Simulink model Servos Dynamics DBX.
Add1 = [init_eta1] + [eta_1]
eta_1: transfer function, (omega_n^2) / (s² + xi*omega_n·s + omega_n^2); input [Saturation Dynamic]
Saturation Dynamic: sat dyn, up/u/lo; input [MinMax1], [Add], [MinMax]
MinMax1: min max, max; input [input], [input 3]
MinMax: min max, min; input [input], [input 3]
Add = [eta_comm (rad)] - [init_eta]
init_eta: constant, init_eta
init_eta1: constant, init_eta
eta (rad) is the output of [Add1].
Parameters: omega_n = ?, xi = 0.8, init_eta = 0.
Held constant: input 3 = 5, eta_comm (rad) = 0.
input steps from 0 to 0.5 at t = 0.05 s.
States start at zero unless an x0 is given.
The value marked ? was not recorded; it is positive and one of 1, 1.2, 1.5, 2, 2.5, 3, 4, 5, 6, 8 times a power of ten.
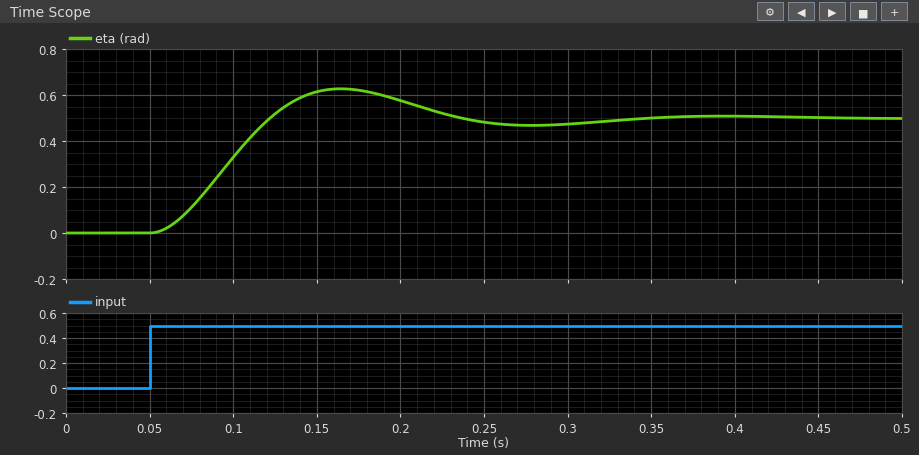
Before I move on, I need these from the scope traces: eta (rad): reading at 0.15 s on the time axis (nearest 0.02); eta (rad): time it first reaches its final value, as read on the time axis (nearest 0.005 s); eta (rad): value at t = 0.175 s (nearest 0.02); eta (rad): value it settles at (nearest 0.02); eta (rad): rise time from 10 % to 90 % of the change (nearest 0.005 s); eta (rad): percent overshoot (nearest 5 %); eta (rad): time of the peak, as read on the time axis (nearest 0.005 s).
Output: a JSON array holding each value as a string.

["0.62", "0.120 s", "0.62", "0.50", "0.050 s", "25 %", "0.165 s"]
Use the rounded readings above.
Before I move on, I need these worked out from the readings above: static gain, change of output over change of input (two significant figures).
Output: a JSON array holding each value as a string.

["1.0"]
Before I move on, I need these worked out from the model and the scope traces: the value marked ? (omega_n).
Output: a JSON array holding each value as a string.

["30"]
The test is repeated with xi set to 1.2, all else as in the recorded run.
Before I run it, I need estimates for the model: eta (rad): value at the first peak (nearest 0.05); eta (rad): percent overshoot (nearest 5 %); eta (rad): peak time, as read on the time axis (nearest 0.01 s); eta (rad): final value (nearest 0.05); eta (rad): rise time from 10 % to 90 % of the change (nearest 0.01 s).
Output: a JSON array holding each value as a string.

["0.55", "10 %", "0.18 s", "0.50", "0.06 s"]
